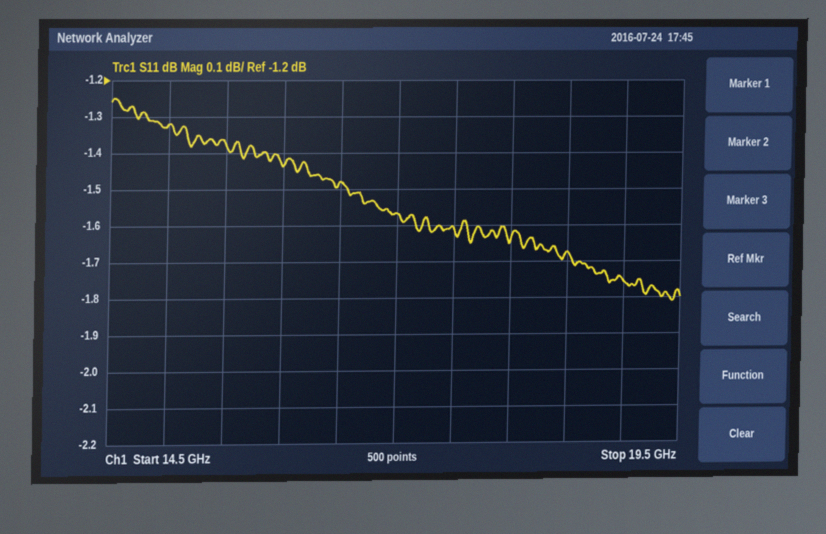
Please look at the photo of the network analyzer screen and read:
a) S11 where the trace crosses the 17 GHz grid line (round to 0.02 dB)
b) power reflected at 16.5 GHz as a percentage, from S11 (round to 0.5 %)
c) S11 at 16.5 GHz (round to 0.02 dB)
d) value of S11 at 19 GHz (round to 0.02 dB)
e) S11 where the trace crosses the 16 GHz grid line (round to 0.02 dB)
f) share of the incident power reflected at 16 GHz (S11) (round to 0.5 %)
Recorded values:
-1.56 dB
71.0 %
-1.48 dB
-1.76 dB
-1.44 dB
72.0 %
